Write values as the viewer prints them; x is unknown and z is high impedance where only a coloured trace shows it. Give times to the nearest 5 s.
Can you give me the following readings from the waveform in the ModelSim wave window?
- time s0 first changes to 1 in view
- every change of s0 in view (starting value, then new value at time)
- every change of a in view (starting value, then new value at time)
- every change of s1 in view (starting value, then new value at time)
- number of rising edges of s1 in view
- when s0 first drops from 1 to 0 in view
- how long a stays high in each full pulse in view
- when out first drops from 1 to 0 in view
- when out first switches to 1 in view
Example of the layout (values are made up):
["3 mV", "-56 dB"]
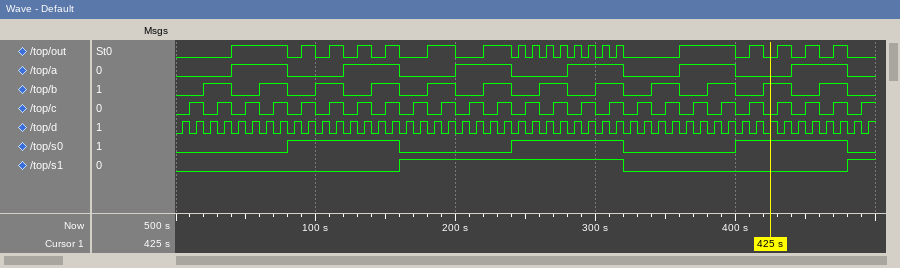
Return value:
["80 s", "0, 1 at 80 s, 0 at 160 s, 1 at 240 s, 0 at 320 s, 1 at 400 s, 0 at 480 s", "0, 1 at 40 s, 0 at 80 s, 1 at 120 s, 0 at 160 s, 1 at 200 s, 0 at 240 s, 1 at 280 s, 0 at 320 s, 1 at 360 s, 0 at 400 s, 1 at 440 s, 0 at 480 s", "0, 1 at 160 s, 0 at 320 s, 1 at 480 s", "2", "160 s", "40 s, 40 s, 40 s, 40 s, 40 s, 40 s", "80 s", "40 s"]
